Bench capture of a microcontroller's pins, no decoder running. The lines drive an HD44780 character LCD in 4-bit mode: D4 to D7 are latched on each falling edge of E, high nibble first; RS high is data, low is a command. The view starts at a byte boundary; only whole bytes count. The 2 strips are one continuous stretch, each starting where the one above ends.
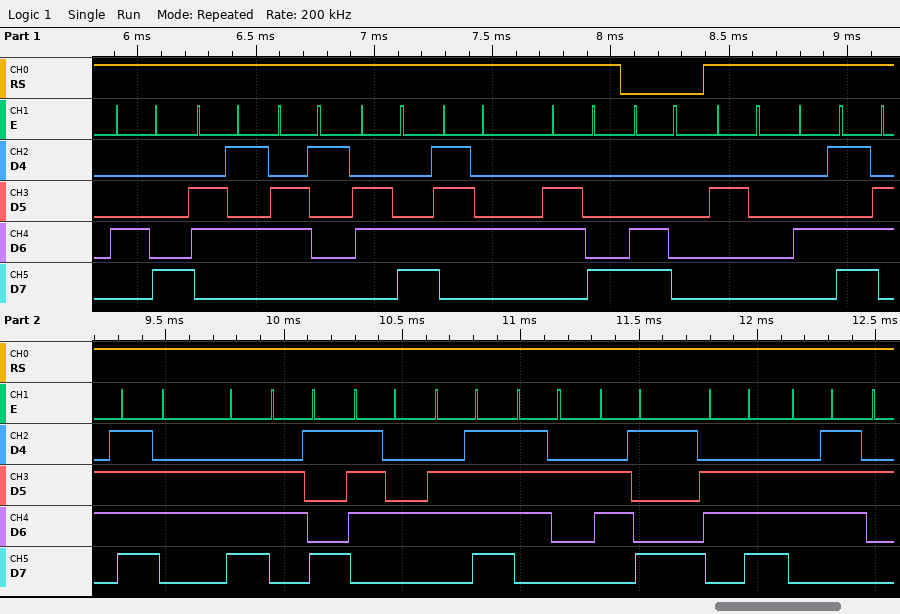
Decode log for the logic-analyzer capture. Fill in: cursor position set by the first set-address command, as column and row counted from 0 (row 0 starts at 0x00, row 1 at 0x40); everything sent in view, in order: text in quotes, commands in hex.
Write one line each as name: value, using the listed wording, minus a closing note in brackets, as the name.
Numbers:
cursor position set by the first set-address command, as column and row counted from 0: column 0, row 1
everything sent in view, in order: text in quotes, commands in hex: "Health" 0xC0 " Monitoring"
